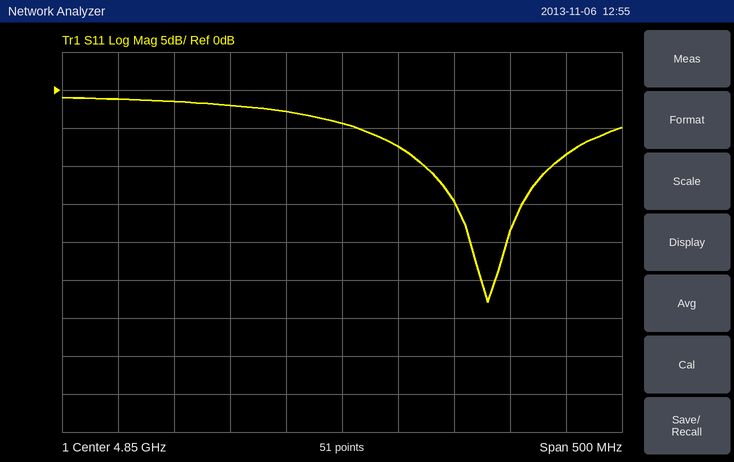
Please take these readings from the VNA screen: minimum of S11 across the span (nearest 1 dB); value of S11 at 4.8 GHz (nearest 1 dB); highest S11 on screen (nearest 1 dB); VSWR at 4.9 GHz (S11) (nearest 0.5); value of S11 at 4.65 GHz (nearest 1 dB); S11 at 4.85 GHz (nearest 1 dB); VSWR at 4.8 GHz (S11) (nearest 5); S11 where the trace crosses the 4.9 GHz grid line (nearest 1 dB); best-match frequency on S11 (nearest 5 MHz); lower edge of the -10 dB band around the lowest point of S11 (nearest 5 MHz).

-28 dB
-3 dB
-1 dB
2.5
-1 dB
-4 dB
5
-7 dB
4.980 GHz
4.925 GHz
